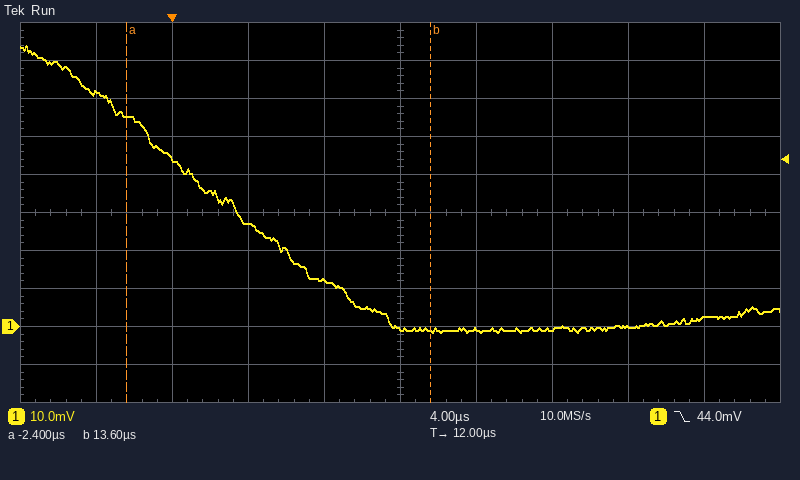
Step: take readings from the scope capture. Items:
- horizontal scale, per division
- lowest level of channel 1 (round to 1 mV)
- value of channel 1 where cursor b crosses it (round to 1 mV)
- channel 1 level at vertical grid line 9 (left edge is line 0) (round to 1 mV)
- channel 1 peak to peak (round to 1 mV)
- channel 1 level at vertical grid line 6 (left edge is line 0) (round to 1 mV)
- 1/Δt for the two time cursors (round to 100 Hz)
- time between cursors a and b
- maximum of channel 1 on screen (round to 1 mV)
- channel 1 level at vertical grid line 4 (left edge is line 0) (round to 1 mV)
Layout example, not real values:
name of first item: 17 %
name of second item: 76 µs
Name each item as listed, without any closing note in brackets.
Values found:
horizontal scale, per division: 4 µs
lowest level of channel 1: -2 mV
value of channel 1 where cursor b crosses it: -1 mV
channel 1 level at vertical grid line 9 (left edge is line 0): 2 mV
channel 1 peak to peak: 76 mV
channel 1 level at vertical grid line 6 (left edge is line 0): -1 mV
1/Δt for the two time cursors: 62.5 kHz
time between cursors a and b: 16.0 µs
maximum of channel 1 on screen: 74 mV
channel 1 level at vertical grid line 4 (left edge is line 0): 12 mV
